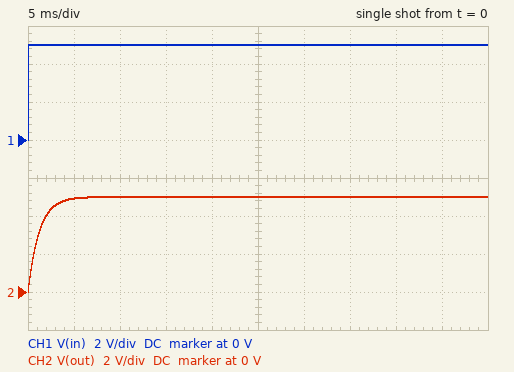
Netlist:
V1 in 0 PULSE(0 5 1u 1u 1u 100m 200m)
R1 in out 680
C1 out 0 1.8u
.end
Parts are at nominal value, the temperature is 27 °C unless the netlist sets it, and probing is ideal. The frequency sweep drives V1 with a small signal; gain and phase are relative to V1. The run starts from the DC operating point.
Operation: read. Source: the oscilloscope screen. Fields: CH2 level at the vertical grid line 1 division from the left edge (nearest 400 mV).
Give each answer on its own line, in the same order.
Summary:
4.8 V
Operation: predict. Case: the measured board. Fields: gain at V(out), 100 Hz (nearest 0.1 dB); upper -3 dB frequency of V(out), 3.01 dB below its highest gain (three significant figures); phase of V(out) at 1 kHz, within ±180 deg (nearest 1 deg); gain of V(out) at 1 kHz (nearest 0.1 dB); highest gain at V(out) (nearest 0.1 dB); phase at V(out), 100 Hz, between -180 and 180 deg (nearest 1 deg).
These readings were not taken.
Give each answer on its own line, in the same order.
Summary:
-2.0 dB
130 Hz
-83 deg
-17.8 dB
0 dB
-38 deg
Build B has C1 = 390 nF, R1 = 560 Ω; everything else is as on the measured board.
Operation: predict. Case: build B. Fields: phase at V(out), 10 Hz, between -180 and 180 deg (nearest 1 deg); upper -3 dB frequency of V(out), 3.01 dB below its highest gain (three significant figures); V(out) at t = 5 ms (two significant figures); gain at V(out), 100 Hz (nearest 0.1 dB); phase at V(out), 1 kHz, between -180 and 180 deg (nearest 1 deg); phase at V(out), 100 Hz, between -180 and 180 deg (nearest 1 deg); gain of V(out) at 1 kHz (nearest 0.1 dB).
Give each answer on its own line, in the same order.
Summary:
-1 deg
729 Hz
5.0 V
-0.1 dB
-54 deg
-8 deg
-4.6 dB
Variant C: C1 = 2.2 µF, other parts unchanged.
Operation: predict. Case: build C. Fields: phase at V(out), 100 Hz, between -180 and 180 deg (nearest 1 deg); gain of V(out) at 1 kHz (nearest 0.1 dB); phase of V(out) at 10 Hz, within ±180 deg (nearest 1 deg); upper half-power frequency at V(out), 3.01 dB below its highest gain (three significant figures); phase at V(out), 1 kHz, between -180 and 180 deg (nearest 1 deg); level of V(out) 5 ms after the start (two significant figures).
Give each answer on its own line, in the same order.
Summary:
-43 deg
-19.5 dB
-5 deg
106 Hz
-84 deg
4.8 V
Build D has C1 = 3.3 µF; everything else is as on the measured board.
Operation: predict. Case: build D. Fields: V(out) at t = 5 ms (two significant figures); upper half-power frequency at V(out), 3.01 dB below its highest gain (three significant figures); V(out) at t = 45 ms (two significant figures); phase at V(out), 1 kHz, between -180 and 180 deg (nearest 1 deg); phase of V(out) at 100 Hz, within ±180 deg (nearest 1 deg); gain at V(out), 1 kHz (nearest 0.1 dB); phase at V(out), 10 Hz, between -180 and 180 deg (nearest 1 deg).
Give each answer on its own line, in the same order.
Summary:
4.5 V
70.9 Hz
5.0 V
-86 deg
-55 deg
-23.0 dB
-8 deg
